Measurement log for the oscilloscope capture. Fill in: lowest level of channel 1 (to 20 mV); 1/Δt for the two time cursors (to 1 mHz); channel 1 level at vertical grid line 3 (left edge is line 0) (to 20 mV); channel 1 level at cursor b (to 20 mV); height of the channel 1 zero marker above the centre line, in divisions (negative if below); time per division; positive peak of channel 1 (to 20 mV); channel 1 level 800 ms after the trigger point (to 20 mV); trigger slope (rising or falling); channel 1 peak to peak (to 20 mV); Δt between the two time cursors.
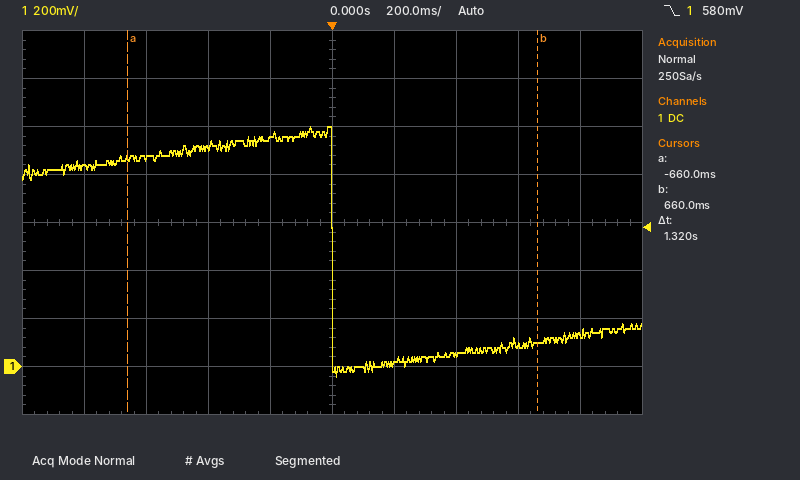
-40 mV
758 mHz
920 mV
100 mV
-3.0 div
200 ms
1.00 V
140 mV
falling
1.04 V
1.32 s
